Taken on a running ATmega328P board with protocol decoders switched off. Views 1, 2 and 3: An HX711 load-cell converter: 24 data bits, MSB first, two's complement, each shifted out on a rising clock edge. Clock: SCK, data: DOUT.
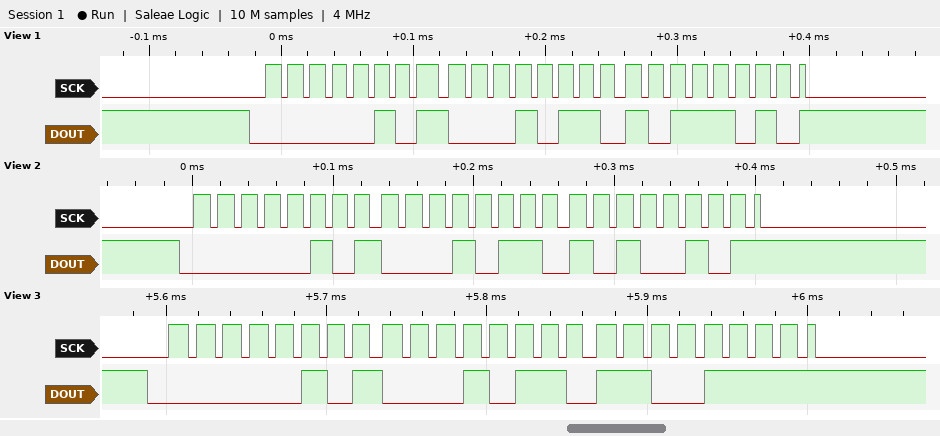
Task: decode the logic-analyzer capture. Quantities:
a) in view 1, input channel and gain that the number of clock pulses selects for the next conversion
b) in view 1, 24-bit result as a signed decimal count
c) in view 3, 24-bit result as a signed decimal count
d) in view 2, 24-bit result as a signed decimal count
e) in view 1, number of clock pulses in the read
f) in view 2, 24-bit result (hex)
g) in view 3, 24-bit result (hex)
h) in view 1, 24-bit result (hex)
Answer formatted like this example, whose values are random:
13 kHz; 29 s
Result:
channel A, gain 128; 333498; 333519; 333477; 25; 0x0516A5; 0x0516CF; 0x0516BA
